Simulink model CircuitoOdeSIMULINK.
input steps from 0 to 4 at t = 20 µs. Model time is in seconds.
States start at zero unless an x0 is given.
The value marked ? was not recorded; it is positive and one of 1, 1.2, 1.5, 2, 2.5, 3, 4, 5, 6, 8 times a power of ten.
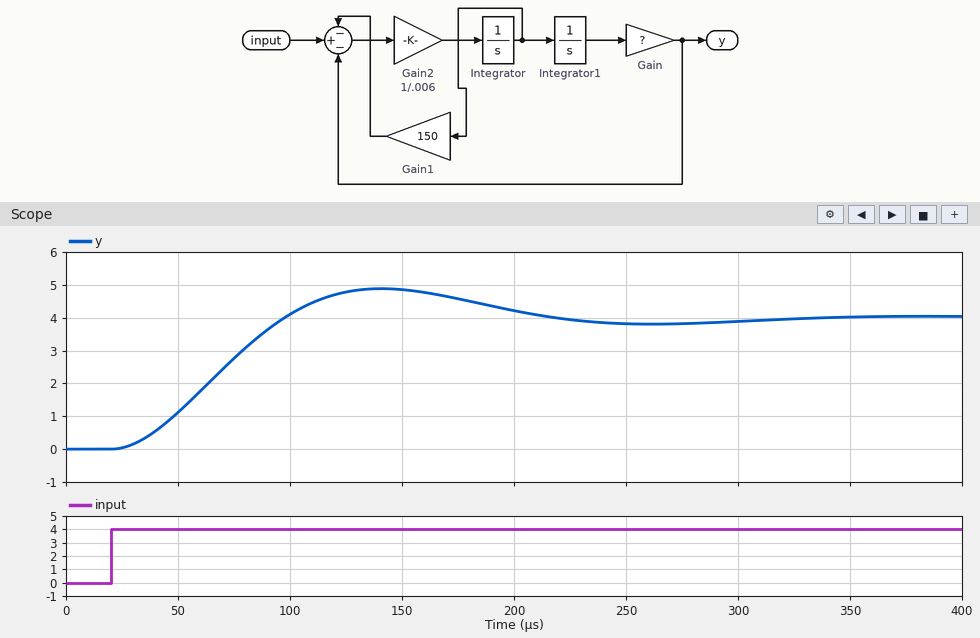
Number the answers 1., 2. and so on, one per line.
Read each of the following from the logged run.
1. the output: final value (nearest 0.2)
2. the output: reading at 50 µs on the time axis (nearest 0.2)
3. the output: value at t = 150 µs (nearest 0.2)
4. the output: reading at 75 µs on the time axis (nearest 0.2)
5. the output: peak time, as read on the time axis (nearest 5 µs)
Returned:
1. 4.0
2. 1.2
3. 4.8
4. 2.8
5. 140 µs
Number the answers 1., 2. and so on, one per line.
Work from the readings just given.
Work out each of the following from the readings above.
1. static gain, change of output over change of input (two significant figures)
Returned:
1. 1.0
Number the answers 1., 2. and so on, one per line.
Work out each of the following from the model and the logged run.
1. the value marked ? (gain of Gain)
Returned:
1. 5e+06
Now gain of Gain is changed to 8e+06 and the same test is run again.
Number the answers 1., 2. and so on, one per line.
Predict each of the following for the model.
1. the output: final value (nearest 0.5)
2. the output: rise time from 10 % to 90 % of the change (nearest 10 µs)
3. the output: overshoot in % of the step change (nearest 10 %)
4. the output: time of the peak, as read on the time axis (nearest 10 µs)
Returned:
1. 4.0
2. 40 µs
3. 30 %
4. 110 µs
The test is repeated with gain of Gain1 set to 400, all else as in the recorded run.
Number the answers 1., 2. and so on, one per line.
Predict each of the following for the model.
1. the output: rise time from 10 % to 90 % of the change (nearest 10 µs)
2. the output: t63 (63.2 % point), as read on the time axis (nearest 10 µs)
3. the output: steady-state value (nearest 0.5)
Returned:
1. 140 µs
2. 100 µs
3. 4.0
